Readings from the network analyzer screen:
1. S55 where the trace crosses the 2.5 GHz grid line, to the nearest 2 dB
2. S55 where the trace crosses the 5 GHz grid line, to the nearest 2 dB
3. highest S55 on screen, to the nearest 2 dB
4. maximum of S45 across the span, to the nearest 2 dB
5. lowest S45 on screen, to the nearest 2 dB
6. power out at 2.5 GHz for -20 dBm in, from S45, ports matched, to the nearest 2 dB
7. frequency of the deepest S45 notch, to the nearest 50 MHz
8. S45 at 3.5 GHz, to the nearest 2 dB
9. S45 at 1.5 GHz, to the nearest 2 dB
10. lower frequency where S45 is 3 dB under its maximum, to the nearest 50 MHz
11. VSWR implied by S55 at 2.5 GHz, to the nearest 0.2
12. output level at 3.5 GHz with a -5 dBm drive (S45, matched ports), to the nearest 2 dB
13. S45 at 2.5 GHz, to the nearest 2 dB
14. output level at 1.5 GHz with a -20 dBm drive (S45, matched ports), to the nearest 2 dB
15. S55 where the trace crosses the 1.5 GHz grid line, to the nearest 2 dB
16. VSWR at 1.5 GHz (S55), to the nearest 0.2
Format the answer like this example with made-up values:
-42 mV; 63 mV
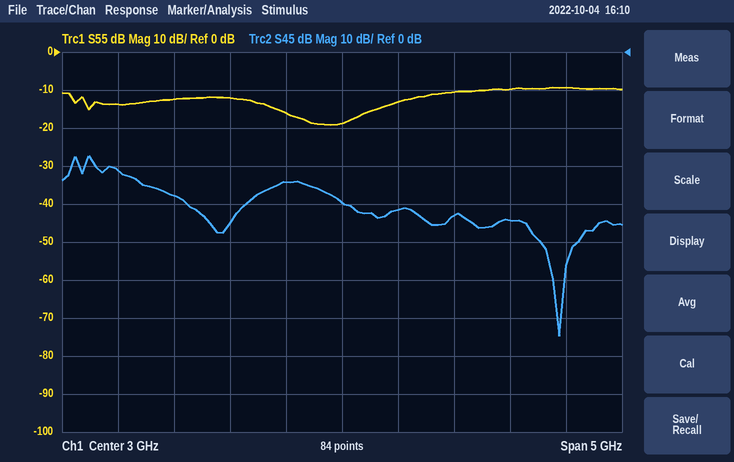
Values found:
-16 dB; -10 dB; -10 dB; -28 dB; -74 dB; -54 dBm; 4.95 GHz; -42 dB; -38 dB; 700 MHz; 1.4; -46 dBm; -34 dB; -58 dBm; -12 dB; 1.6
